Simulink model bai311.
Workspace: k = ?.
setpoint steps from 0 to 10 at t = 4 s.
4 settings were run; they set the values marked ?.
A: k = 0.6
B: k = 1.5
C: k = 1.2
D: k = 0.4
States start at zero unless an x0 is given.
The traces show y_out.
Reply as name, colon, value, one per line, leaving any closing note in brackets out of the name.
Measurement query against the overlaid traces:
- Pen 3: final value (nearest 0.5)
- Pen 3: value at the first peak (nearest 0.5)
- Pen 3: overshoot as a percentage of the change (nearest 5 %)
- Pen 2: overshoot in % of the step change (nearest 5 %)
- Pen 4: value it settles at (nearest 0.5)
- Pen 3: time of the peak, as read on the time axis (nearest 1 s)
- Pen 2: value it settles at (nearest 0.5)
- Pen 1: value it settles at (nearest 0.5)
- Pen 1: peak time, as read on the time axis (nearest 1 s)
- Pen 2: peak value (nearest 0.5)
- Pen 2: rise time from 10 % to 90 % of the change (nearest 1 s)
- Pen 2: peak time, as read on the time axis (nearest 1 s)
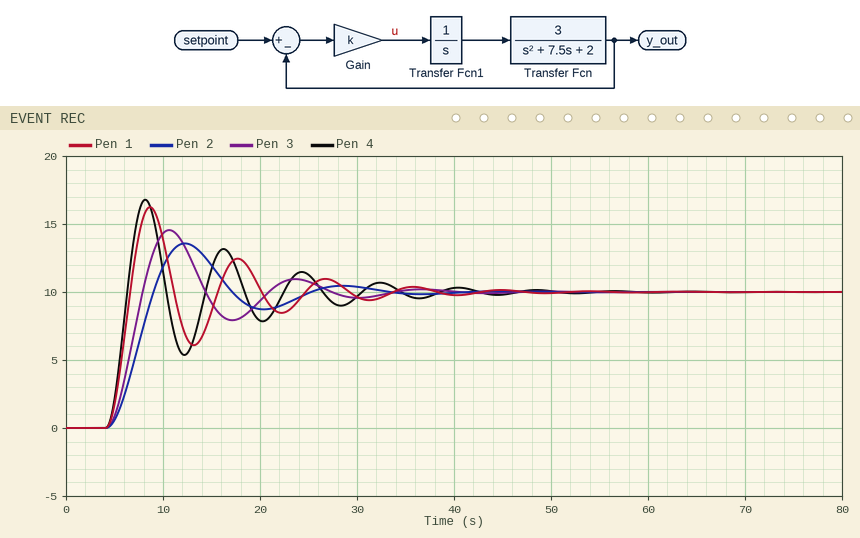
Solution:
Pen 3: final value: 10.0
Pen 3: value at the first peak: 14.5
Pen 3: overshoot as a percentage of the change: 45 %
Pen 2: overshoot in % of the step change: 35 %
Pen 4: value it settles at: 10.0
Pen 3: time of the peak, as read on the time axis: 11 s
Pen 2: value it settles at: 10.0
Pen 1: value it settles at: 10.0
Pen 1: peak time, as read on the time axis: 9 s
Pen 2: peak value: 13.5
Pen 2: rise time from 10 % to 90 % of the change: 3 s
Pen 2: peak time, as read on the time axis: 12 s
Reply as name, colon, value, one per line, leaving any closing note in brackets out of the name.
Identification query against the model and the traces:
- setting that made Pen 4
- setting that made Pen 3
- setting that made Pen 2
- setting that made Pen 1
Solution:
setting that made Pen 4: B
setting that made Pen 3: A
setting that made Pen 2: D
setting that made Pen 1: C
